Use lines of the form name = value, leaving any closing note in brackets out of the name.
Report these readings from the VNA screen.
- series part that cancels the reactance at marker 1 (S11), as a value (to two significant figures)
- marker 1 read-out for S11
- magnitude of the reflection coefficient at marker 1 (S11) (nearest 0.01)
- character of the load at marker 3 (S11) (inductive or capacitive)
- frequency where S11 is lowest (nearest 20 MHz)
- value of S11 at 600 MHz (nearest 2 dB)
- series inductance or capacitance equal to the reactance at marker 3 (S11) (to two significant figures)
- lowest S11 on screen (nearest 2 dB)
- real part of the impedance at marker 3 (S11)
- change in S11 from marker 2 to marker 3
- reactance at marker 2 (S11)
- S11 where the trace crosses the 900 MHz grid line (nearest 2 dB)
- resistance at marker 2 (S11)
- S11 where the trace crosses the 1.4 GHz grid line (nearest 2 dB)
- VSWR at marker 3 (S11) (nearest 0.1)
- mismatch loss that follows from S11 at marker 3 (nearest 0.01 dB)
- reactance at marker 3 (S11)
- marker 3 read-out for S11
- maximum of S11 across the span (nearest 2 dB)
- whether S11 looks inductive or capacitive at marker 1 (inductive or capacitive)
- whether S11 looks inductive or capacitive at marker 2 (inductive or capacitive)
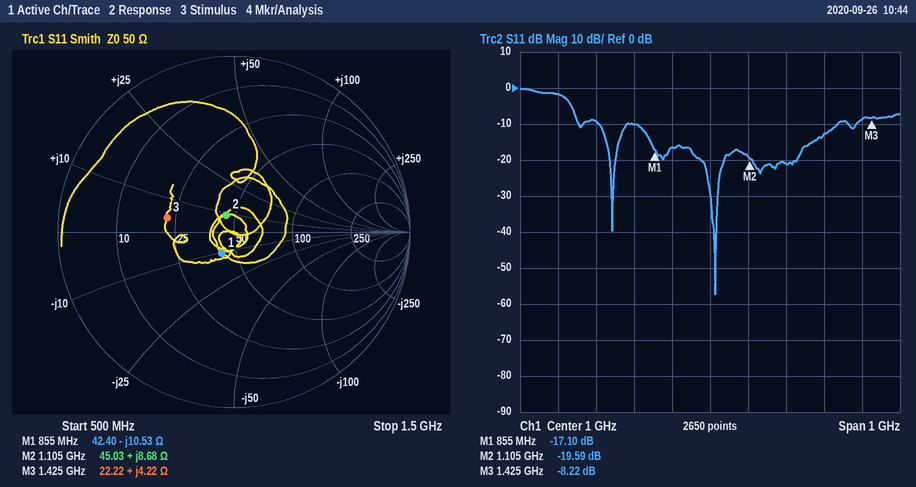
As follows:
series part that cancels the reactance at marker 1 (S11), as a value = 2.0 nH
marker 1 read-out for S11 = -17.10 dB
magnitude of the reflection coefficient at marker 1 (S11) = 0.14
character of the load at marker 3 (S11) = inductive
frequency where S11 is lowest = 1.02 GHz
value of S11 at 600 MHz = -2 dB
series inductance or capacitance equal to the reactance at marker 3 (S11) = 470 pH
lowest S11 on screen = -58 dB
real part of the impedance at marker 3 = 22.22 Ω
change in S11 from marker 2 to marker 3 = 11.37 dB
reactance at marker 2 = +8.68 Ω
S11 where the trace crosses the 900 MHz grid line = -16 dB
resistance at marker 2 = 45.03 Ω
S11 where the trace crosses the 1.4 GHz grid line = -8 dB
VSWR at marker 3 (S11) = 2.3
mismatch loss that follows from S11 at marker 3 = 0.71 dB
reactance at marker 3 = +4.22 Ω
marker 3 read-out for S11 = -8.22 dB
maximum of S11 across the span = 0 dB
whether S11 looks inductive or capacitive at marker 1 = capacitive
whether S11 looks inductive or capacitive at marker 2 = inductive
